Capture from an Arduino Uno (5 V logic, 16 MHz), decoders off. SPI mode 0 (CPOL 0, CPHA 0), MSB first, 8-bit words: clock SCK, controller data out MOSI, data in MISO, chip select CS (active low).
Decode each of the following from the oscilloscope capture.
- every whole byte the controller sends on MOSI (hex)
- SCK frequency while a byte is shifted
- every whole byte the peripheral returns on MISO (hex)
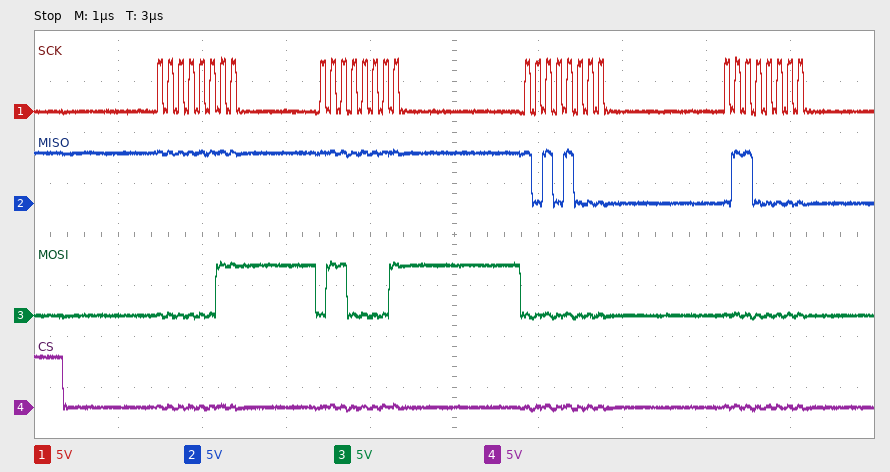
03 61 00 00
8 MHz
FF FF A8 60
